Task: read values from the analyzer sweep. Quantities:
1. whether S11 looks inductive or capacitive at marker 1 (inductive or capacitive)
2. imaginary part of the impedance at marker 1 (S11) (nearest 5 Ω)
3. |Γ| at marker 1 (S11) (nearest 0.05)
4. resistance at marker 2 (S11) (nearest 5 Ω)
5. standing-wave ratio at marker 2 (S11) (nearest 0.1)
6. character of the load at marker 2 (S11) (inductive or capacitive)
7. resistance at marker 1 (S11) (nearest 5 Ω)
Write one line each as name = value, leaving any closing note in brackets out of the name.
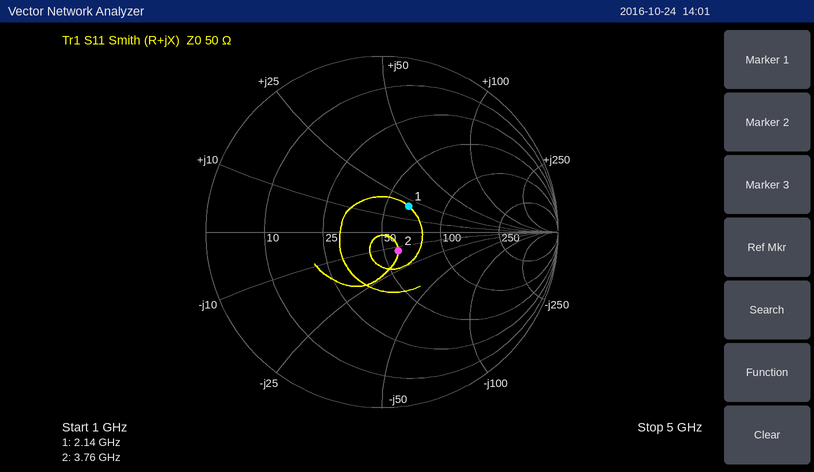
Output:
whether S11 looks inductive or capacitive at marker 1 = inductive
imaginary part of the impedance at marker 1 (S11) = +20 Ω
|Γ| at marker 1 (S11) = 0.20
resistance at marker 2 (S11) = 60 Ω
standing-wave ratio at marker 2 (S11) = 1.3
character of the load at marker 2 (S11) = capacitive
resistance at marker 1 (S11) = 65 Ω
